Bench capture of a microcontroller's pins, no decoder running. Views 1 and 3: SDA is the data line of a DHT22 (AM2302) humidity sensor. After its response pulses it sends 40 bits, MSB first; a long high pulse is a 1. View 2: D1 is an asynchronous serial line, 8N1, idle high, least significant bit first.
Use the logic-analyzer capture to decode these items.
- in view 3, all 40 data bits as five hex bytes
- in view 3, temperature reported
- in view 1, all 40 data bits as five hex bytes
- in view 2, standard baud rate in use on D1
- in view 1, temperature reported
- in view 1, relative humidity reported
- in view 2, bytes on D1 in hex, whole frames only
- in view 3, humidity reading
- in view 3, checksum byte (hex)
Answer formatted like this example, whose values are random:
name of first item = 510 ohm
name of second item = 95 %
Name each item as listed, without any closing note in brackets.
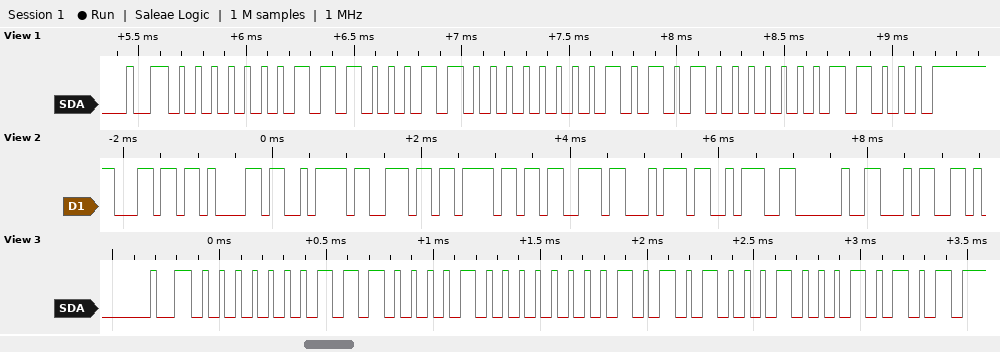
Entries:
in view 3, all 40 data bits as five hex bytes = 01 C2 01 51 15
in view 3, temperature reported = 33.7 °C
in view 1, all 40 data bits as five hex bytes = 01 C6 01 50 18
in view 2, standard baud rate in use on D1 = 9600 baud
in view 1, temperature reported = 33.6 °C
in view 1, relative humidity reported = 45.4 %
in view 2, bytes on D1 in hex, whole frames only = 6C 61 7A 6E 6F 73 74 3A 20 34
in view 3, humidity reading = 45.0 %
in view 3, checksum byte = 0x15
